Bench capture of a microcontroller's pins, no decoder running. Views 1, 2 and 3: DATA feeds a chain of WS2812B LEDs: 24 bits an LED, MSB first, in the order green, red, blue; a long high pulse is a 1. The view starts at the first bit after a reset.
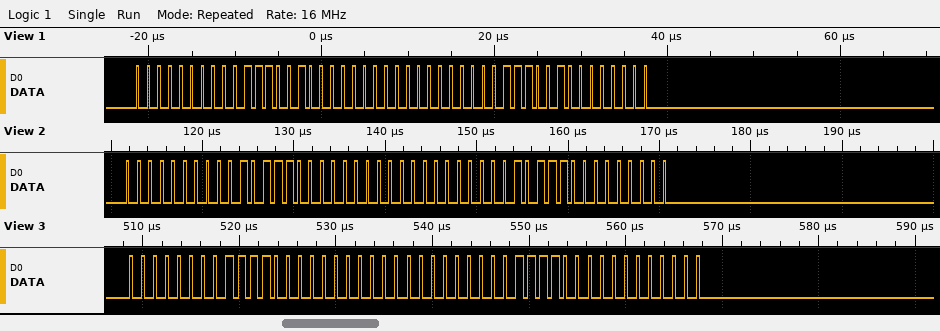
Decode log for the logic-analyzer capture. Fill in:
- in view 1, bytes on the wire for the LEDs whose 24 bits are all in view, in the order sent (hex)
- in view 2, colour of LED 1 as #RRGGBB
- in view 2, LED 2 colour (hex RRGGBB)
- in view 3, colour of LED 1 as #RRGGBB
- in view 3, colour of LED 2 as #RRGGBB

00 39 00 00 39 00
#2E0000
#2E0000
#F00000
#F00000
